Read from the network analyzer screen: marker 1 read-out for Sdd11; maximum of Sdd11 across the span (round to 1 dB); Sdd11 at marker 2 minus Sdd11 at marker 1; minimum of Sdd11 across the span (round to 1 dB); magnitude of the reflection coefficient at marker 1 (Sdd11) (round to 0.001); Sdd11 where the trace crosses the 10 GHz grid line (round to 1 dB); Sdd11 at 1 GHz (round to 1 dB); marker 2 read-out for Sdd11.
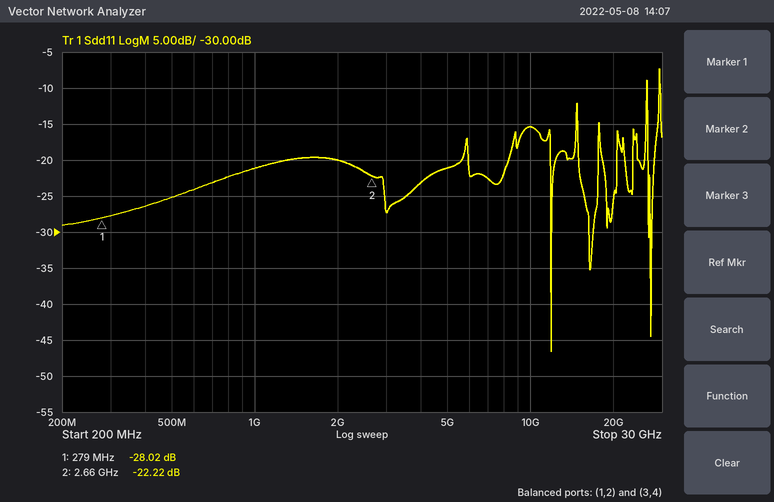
-28.02 dB
-7 dB
5.80 dB
-47 dB
0.040
-15 dB
-21 dB
-22.22 dB
